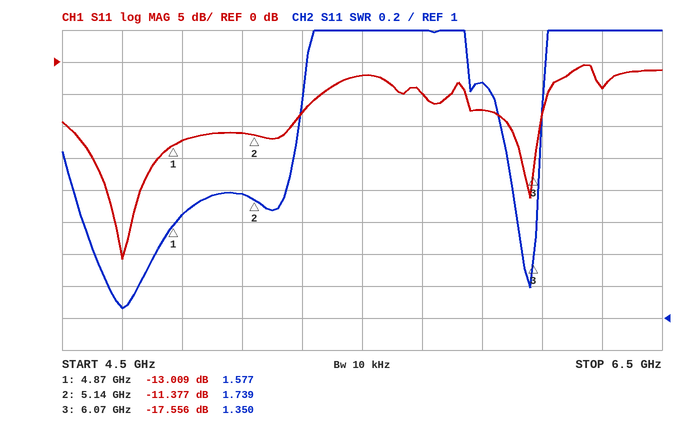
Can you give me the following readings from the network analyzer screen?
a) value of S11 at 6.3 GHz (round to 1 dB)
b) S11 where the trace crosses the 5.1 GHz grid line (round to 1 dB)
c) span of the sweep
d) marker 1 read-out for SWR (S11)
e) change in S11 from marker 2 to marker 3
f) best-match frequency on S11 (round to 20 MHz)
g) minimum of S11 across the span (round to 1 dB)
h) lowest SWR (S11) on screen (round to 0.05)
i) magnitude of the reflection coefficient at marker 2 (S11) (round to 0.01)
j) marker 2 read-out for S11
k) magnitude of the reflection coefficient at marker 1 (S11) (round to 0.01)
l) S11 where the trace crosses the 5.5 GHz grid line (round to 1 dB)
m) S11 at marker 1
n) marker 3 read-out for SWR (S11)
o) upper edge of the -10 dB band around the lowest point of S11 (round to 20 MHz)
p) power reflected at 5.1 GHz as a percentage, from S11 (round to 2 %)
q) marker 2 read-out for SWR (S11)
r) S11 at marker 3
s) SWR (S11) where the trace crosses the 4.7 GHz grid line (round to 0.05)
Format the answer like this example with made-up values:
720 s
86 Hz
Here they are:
-4 dB
-11 dB
2 GHz
1.577
-6.179 dB
4.70 GHz
-31 dB
1.05
0.27
-11.377 dB
0.22
-2 dB
-13.009 dB
1.350
5.26 GHz
8 %
1.739
-17.556 dB
1.05
